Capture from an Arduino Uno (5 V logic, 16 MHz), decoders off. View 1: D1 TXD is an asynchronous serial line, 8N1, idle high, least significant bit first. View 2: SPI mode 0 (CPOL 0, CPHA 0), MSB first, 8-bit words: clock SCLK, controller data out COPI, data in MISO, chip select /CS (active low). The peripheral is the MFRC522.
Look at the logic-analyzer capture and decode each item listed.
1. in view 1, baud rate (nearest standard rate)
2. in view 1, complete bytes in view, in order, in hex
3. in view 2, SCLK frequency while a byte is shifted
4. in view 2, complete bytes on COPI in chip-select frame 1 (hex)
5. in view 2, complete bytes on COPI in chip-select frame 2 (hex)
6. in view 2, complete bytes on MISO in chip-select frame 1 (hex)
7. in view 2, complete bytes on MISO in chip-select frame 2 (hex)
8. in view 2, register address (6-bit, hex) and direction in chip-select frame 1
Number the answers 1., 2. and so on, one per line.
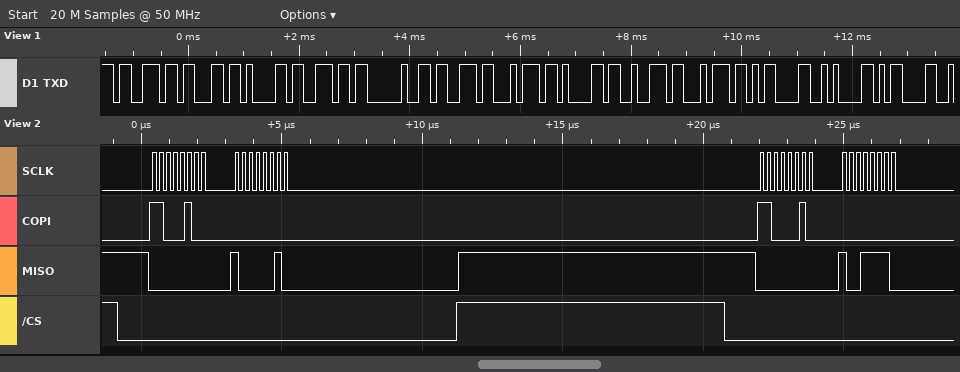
1. 9600 baud
2. 73 63 61 6E 20 73 74 61 72 74 0D 0A 0D
3. 4 MHz
4. 0xC4 0x00
5. 0xC2 0x00
6. 0x00 0x82
7. 0x00 0x9E
8. 0x22 read
